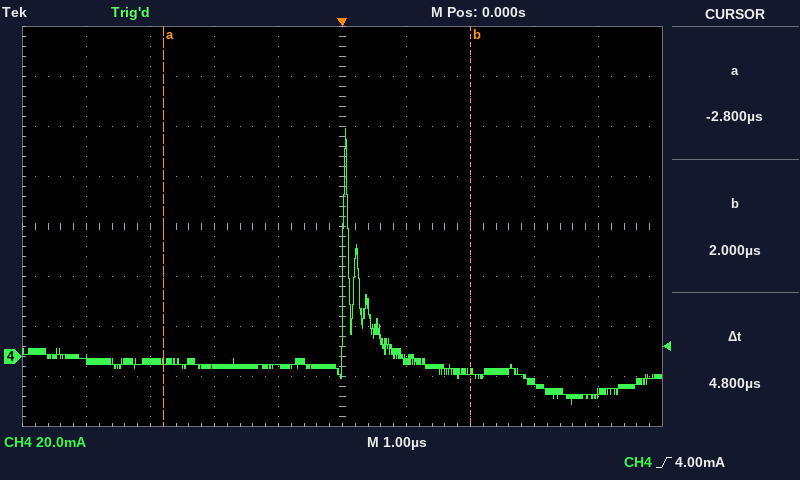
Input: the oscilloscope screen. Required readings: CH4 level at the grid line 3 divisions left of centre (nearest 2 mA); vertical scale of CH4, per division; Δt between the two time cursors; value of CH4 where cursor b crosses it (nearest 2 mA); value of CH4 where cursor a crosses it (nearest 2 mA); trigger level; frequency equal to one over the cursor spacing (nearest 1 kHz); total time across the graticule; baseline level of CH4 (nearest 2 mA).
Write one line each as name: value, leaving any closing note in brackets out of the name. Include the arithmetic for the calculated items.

CH4 level at the grid line 3 divisions left of centre: -2 mA
vertical scale of CH4, per division: 20 mA
Δt between the two time cursors: 4.8 µs
value of CH4 where cursor b crosses it: -6 mA
value of CH4 where cursor a crosses it: -2 mA
trigger level: 4.00 mA
frequency equal to one over the cursor spacing: 1 / 4.8 µs ≈ 208 kHz
total time across the graticule: 10 µs
baseline level of CH4: -4 mA
